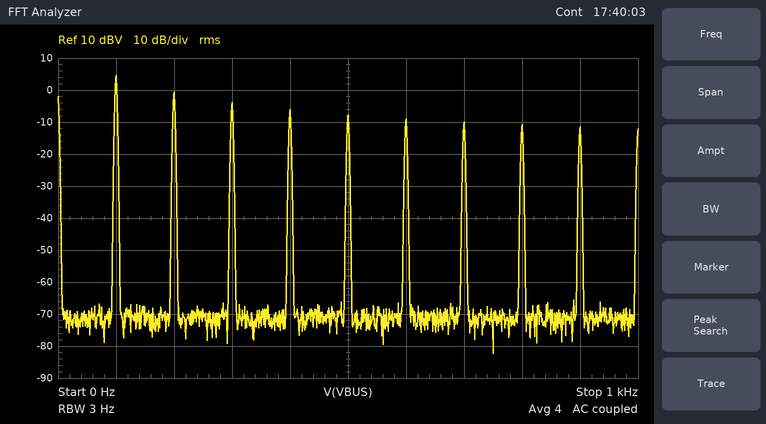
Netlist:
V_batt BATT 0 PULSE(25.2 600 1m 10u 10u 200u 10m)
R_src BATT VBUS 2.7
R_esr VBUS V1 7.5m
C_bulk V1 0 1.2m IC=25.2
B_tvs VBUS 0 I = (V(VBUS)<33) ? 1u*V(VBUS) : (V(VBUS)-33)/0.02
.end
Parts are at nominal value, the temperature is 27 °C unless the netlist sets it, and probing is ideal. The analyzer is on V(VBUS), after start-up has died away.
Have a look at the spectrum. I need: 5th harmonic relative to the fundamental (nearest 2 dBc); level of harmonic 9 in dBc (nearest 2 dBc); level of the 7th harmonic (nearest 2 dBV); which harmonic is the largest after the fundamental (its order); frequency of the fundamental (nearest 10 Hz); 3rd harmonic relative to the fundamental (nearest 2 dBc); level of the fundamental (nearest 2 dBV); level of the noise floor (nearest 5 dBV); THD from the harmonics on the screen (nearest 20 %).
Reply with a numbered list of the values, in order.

1. -12 dBc
2. -16 dBc
3. -10 dBV
4. 2
5. 100 Hz
6. -8 dBc
7. 4 dBV
8. -70 dBV
9. 80 %
